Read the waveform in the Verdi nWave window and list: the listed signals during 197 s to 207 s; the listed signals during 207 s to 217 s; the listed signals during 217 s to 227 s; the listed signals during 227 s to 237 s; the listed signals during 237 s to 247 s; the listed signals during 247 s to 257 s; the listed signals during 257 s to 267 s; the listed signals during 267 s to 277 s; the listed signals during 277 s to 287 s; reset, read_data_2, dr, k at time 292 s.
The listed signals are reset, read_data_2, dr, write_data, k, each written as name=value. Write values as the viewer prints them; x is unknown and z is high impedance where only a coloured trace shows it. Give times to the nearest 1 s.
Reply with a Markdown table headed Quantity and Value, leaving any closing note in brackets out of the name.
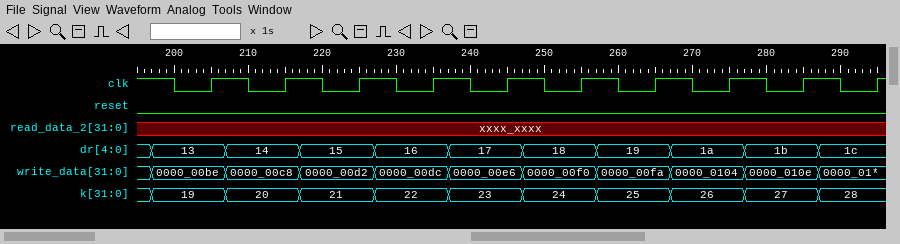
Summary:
| Quantity | Value |
|---|---|
| the listed signals during 197 s to 207 s | reset=0, read_data_2=xxxx_xxxx, dr=13, write_data=0000_00be, k=19 |
| the listed signals during 207 s to 217 s | reset=0, read_data_2=xxxx_xxxx, dr=14, write_data=0000_00c8, k=20 |
| the listed signals during 217 s to 227 s | reset=0, read_data_2=xxxx_xxxx, dr=15, write_data=0000_00d2, k=21 |
| the listed signals during 227 s to 237 s | reset=0, read_data_2=xxxx_xxxx, dr=16, write_data=0000_00dc, k=22 |
| the listed signals during 237 s to 247 s | reset=0, read_data_2=xxxx_xxxx, dr=17, write_data=0000_00e6, k=23 |
| the listed signals during 247 s to 257 s | reset=0, read_data_2=xxxx_xxxx, dr=18, write_data=0000_00f0, k=24 |
| the listed signals during 257 s to 267 s | reset=0, read_data_2=xxxx_xxxx, dr=19, write_data=0000_00fa, k=25 |
| the listed signals during 267 s to 277 s | reset=0, read_data_2=xxxx_xxxx, dr=1a, write_data=0000_0104, k=26 |
| the listed signals during 277 s to 287 s | reset=0, read_data_2=xxxx_xxxx, dr=1b, write_data=0000_010e, k=27 |
| reset, read_data_2, dr, k at time 292 s | reset=0, read_data_2=xxxx_xxxx, dr=1c, k=28 |
